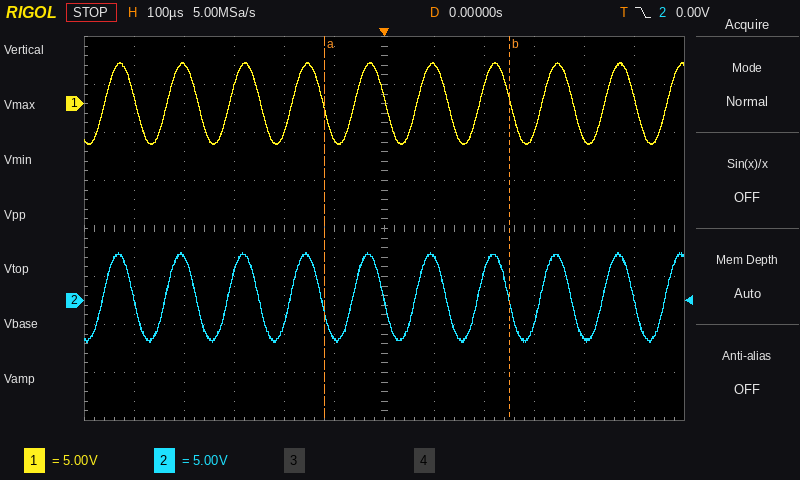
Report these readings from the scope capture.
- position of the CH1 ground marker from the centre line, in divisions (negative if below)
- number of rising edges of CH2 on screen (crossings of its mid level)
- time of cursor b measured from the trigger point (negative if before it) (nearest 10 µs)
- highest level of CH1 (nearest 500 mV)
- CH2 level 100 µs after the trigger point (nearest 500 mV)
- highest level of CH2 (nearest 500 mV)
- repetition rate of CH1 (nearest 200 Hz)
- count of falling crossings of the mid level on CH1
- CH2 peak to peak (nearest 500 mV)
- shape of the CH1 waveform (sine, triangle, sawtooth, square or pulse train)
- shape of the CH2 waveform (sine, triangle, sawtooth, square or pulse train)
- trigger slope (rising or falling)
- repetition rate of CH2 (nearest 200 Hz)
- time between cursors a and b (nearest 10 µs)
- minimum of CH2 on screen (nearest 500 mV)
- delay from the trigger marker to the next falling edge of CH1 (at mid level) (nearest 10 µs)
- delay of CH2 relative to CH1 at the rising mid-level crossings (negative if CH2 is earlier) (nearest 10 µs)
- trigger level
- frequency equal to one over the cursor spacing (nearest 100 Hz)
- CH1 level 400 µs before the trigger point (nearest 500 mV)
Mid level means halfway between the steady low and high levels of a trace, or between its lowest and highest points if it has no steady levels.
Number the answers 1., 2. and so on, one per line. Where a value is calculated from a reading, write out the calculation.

1. +2.6 div
2. 10
3. +250 µs
4. 4.5 V
5. 4.5 V
6. 5.0 V
7. 8.0 kHz
8. 9
9. 5.0 V − (-4.5 V) = 9.5 V
10. sine
11. sine
12. falling
13. 8.0 kHz
14. 370 µs
15. -4.5 V
16. 130 µs
17. 0 µs
18. 0.00 V
19. 1 / 370 µs ≈ 2.7 kHz
20. 4.0 V
